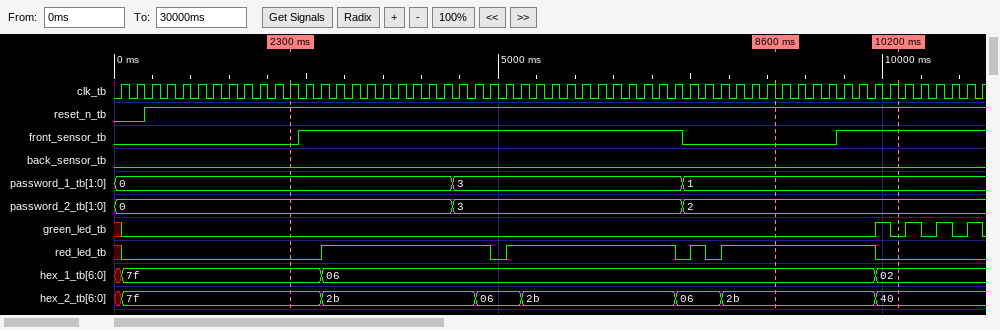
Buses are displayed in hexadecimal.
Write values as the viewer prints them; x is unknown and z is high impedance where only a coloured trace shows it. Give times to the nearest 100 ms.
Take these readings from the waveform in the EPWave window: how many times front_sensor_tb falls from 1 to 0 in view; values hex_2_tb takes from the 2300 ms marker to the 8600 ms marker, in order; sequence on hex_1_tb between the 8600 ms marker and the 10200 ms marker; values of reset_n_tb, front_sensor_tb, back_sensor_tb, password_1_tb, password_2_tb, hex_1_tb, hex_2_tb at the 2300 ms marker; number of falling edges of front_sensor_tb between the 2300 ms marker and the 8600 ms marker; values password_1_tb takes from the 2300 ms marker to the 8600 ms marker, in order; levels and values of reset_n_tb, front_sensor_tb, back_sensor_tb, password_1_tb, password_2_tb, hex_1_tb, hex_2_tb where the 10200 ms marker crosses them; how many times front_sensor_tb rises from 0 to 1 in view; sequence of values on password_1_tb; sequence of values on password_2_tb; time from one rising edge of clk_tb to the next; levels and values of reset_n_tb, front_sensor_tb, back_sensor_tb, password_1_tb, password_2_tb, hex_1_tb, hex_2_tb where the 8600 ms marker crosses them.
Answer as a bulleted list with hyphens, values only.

- 1
- 7f, 2b, 06, 2b, 06, 2b
- 06, 02
- reset_n_tb=1, front_sensor_tb=0, back_sensor_tb=0, password_1_tb=0, password_2_tb=0, hex_1_tb=7f, hex_2_tb=7f
- 1
- 0, 3, 1
- reset_n_tb=1, front_sensor_tb=1, back_sensor_tb=0, password_1_tb=1, password_2_tb=2, hex_1_tb=02, hex_2_tb=40
- 2
- 0, 3, 1
- 0, 3, 2
- 200 ms
- reset_n_tb=1, front_sensor_tb=0, back_sensor_tb=0, password_1_tb=1, password_2_tb=2, hex_1_tb=06, hex_2_tb=2b
